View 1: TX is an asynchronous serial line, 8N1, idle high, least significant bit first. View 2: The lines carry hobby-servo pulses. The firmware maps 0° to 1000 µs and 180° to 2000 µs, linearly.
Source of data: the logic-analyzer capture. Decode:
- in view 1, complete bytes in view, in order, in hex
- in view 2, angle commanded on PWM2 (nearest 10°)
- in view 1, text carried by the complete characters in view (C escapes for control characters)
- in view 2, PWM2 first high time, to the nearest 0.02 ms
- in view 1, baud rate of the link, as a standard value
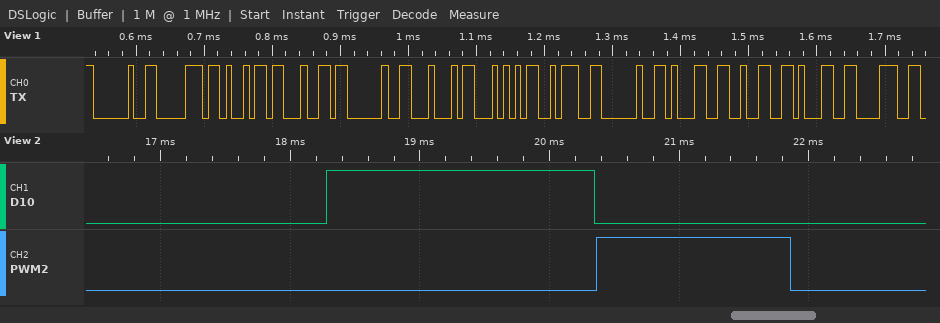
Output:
20 70 69 64 20 44 54 3A 20 31 32 31 38
90°
" pid DT: 1218"
1.50 ms
115200 baud
